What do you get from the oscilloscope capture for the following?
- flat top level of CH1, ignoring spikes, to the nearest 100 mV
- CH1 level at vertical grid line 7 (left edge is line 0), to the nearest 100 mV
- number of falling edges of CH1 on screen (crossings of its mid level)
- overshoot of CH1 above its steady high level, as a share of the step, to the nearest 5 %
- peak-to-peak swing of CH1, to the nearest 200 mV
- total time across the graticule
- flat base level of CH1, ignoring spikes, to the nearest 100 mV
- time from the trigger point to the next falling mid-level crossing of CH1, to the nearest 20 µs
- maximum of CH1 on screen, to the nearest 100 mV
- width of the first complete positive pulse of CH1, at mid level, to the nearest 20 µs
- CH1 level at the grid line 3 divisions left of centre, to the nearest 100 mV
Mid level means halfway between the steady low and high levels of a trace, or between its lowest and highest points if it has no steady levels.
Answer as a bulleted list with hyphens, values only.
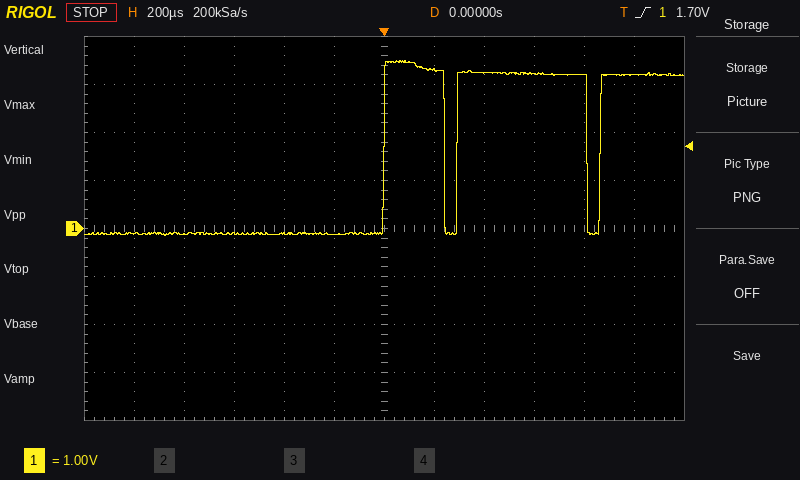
- 3.2 V
- 3.3 V
- 2
- 10 %
- 3.6 V
- 2.4 ms
- -100 mV
- 240 µs
- 3.5 V
- 240 µs
- -100 mV
